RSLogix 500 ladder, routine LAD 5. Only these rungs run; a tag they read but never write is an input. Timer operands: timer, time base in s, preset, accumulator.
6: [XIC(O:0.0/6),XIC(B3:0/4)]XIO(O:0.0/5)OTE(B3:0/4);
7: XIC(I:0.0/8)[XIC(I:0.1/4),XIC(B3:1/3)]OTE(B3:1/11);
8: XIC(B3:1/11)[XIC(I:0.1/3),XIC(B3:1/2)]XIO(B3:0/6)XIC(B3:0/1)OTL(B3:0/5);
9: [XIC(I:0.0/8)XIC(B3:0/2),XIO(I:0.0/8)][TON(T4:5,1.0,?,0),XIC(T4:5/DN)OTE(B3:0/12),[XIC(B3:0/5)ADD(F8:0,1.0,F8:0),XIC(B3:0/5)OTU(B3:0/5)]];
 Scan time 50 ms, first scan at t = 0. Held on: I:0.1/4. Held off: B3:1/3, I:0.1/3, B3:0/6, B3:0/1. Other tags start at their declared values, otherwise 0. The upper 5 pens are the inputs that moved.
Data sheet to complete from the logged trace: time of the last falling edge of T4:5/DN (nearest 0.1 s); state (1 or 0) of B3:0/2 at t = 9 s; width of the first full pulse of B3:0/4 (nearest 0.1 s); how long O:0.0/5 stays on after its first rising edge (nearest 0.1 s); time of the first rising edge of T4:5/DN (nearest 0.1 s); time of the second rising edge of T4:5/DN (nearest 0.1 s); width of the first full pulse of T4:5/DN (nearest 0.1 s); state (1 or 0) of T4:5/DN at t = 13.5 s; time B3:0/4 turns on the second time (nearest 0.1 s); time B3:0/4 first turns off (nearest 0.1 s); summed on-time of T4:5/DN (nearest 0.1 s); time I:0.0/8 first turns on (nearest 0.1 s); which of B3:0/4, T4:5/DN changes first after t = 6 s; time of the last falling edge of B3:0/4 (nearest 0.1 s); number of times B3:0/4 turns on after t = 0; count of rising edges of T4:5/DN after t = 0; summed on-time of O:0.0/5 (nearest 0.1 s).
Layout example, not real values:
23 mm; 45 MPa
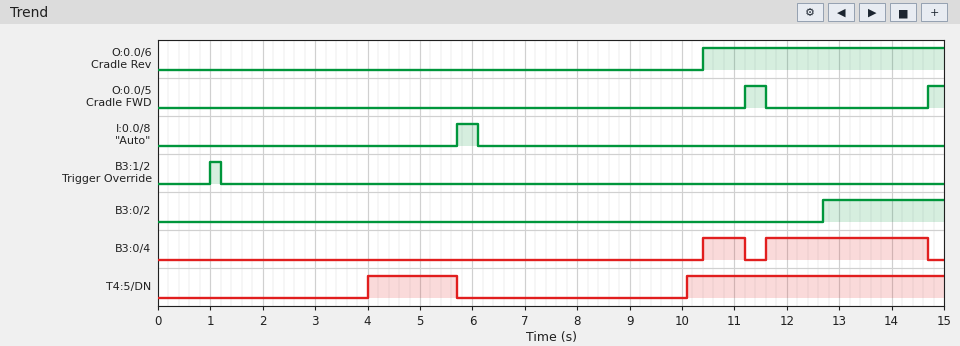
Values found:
5.7 s; 0; 0.8 s; 0.4 s; 4.0 s; 10.1 s; 1.7 s; 1; 11.6 s; 11.2 s; 6.6 s; 5.7 s; T4:5/DN; 14.7 s; 2; 2; 0.7 s
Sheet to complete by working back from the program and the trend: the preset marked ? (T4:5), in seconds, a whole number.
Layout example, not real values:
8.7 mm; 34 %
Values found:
4 s
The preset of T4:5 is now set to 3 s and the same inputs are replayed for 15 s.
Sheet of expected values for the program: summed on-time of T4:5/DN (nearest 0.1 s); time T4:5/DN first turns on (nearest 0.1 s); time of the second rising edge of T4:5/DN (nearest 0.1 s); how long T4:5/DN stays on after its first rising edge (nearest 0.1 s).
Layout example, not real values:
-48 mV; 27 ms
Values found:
8.6 s; 3.0 s; 9.1 s; 2.7 s
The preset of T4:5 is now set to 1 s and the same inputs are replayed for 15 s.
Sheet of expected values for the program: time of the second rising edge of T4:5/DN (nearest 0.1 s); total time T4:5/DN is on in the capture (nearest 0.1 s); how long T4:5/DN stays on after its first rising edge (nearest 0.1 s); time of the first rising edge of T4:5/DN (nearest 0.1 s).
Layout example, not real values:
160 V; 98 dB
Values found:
7.1 s; 12.6 s; 4.7 s; 1.0 s
